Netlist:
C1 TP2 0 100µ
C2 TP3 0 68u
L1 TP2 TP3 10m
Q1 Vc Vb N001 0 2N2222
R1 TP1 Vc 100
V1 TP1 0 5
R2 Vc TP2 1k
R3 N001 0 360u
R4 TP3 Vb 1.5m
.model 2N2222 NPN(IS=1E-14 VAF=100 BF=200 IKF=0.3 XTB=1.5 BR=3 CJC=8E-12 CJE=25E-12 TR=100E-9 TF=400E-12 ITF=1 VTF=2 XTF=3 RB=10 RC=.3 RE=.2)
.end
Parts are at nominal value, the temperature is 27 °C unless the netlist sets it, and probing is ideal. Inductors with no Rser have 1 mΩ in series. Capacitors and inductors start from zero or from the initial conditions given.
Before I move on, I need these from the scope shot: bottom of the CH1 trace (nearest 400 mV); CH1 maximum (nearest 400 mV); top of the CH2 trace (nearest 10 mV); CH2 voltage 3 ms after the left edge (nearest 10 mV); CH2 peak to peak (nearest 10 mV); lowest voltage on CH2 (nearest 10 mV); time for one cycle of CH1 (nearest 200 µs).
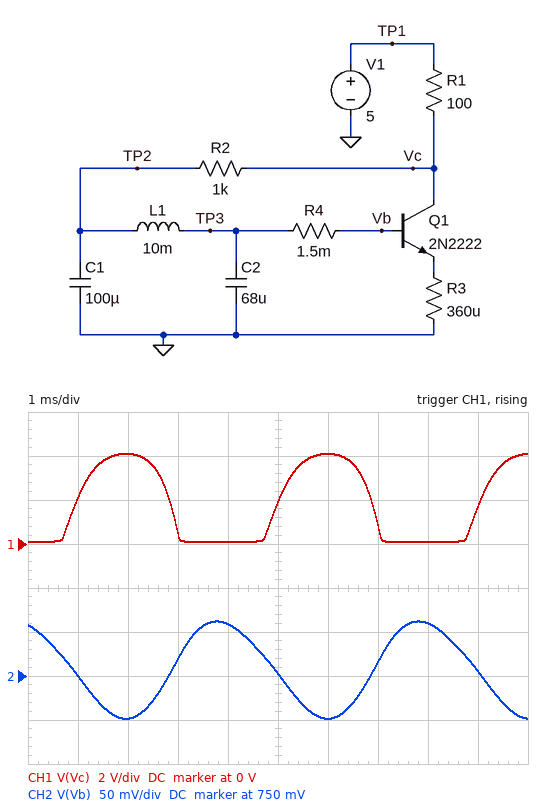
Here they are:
0 V
4.0 V
810 mV
770 mV
110 mV
700 mV
4.0 ms
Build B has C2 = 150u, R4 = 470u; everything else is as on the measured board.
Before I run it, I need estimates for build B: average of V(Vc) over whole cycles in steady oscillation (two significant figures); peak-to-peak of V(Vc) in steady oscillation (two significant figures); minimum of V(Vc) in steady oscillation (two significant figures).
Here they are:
2.7 V
4.6 V
62 mV
